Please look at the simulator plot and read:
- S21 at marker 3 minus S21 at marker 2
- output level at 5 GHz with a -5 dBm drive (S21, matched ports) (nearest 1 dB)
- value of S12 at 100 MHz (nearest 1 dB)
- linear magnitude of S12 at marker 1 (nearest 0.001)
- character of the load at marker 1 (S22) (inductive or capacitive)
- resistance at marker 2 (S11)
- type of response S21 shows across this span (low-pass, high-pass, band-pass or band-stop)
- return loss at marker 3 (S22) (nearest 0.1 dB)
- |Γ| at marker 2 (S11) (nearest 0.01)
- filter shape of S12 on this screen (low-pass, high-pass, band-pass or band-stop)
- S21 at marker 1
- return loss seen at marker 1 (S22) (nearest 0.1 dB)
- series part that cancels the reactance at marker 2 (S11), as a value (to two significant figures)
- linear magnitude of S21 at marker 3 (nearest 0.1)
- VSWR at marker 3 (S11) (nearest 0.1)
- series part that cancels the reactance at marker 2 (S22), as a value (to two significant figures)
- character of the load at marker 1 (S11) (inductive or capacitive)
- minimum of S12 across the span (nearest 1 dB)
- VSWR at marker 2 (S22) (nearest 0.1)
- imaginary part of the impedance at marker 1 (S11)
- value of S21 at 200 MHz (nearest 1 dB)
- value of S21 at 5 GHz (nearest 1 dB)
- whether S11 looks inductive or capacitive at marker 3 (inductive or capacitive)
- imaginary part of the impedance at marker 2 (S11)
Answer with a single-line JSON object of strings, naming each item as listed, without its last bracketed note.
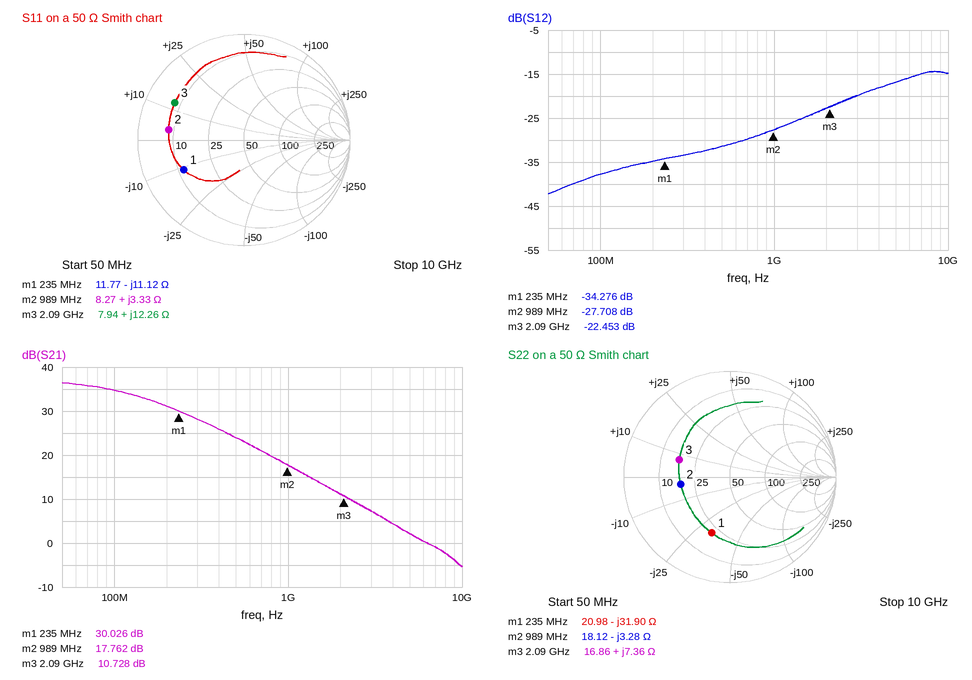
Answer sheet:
{"S21 at marker 3 minus S21 at marker 2": "-7.034 dB", "output level at 5 GHz with a -5 dBm drive (S21, matched ports)": "-3 dBm", "value of S12 at 100 MHz": "-38 dB", "linear magnitude of S12 at marker 1": "0.019", "character of the load at marker 1 (S22)": "capacitive", "resistance at marker 2": "8.27 Ω", "type of response S21 shows across this span": "low-pass", "return loss at marker 3 (S22)": "5.9 dB", "|Γ| at marker 2 (S11)": "0.72", "filter shape of S12 on this screen": "high-pass", "S21 at marker 1": "30.026 dB", "return loss seen at marker 1 (S22)": "5.1 dB", "series part that cancels the reactance at marker 2 (S11), as a value": "48 pF", "linear magnitude of S21 at marker 3": "3.4", "VSWR at marker 3 (S11)": "6.7", "series part that cancels the reactance at marker 2 (S22), as a value": "530 pH", "character of the load at marker 1 (S11)": "capacitive", "minimum of S12 across the span": "-42 dB", "VSWR at marker 2 (S22)": "2.8", "imaginary part of the impedance at marker 1": "-11.12 Ω", "value of S21 at 200 MHz": "31 dB", "value of S21 at 5 GHz": "2 dB", "whether S11 looks inductive or capacitive at marker 3": "inductive", "imaginary part of the impedance at marker 2": "+3.33 Ω"}
